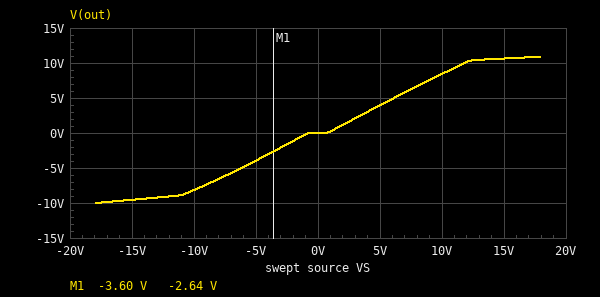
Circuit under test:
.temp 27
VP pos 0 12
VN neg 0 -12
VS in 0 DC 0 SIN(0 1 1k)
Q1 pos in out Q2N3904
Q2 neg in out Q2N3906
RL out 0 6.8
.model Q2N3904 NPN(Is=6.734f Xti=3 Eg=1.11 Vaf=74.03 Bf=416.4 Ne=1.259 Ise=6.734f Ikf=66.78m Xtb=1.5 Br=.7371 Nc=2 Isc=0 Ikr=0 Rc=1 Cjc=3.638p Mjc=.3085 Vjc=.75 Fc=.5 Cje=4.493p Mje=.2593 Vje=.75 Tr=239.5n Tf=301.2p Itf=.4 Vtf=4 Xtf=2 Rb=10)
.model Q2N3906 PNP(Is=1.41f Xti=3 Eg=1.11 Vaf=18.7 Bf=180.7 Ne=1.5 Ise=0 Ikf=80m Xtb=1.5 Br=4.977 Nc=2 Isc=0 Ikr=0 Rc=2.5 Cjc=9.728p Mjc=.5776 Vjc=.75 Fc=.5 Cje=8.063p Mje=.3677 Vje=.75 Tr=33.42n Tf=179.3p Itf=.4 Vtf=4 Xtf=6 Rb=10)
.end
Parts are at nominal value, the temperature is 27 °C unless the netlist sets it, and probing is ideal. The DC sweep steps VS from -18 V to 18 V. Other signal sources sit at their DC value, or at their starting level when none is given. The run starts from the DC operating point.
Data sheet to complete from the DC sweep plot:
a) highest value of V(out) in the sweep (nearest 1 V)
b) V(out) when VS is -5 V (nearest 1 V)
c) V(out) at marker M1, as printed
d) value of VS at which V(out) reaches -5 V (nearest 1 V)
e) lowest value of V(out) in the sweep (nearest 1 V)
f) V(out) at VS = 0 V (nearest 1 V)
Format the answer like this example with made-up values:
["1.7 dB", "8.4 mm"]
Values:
["11 V", "-4 V", "-2.64 V", "-6 V", "-10 V", "0 V"]
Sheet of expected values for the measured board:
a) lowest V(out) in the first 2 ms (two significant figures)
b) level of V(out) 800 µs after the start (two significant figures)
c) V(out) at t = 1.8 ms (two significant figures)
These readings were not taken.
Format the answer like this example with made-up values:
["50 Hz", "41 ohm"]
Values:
["-210 mV", "-170 mV", "-170 mV"]
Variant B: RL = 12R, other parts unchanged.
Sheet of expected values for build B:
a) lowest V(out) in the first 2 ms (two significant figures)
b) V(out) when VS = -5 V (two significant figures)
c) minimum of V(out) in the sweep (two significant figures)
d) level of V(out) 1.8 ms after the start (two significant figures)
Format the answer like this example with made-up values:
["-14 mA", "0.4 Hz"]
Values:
["-230 mV", "-4.1 V", "-11 V", "-180 mV"]
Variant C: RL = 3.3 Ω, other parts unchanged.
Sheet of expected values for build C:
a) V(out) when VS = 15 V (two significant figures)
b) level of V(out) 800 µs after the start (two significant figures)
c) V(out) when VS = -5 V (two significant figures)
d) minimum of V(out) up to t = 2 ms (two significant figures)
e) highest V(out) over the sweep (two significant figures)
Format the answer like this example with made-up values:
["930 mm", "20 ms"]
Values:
["9.4 V", "-150 mV", "-3.6 V", "-190 mV", "9.7 V"]
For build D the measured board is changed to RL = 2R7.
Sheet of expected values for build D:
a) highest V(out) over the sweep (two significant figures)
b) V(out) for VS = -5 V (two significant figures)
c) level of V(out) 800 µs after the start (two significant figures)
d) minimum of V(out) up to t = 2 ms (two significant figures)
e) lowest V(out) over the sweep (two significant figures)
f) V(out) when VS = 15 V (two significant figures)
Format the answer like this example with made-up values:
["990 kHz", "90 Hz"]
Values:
["9.2 V", "-3.4 V", "-140 mV", "-180 mV", "-7.4 V", "9.0 V"]
